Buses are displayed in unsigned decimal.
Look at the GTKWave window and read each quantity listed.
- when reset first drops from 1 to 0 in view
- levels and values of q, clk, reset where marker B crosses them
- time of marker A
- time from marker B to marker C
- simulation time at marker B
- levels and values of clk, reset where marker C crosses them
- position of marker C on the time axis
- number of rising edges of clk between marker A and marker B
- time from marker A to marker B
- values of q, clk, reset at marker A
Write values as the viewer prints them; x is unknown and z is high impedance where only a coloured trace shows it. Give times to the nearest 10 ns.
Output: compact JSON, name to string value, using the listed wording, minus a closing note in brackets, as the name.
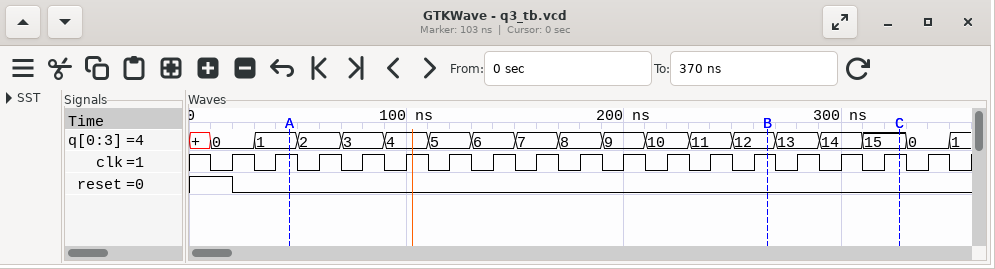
{"when reset first drops from 1 to 0 in view": "20 ns", "levels and values of q, clk, reset where marker B crosses them": "q=12, clk=1, reset=0", "time of marker A": "50 ns", "time from marker B to marker C": "60 ns", "simulation time at marker B": "270 ns", "levels and values of clk, reset where marker C crosses them": "clk=1, reset=0", "position of marker C on the time axis": "330 ns", "number of rising edges of clk between marker A and marker B": "11", "time from marker A to marker B": "220 ns", "values of q, clk, reset at marker A": "q=1, clk=1, reset=0"}
